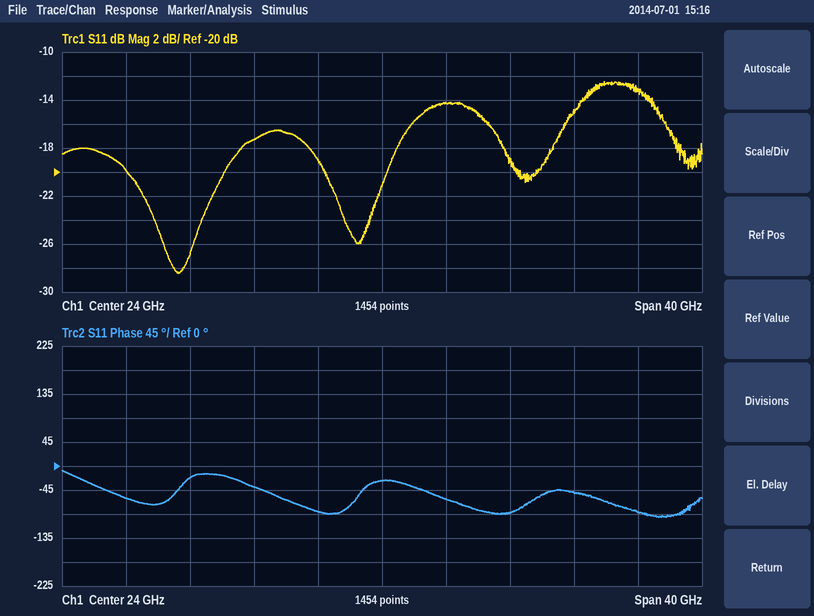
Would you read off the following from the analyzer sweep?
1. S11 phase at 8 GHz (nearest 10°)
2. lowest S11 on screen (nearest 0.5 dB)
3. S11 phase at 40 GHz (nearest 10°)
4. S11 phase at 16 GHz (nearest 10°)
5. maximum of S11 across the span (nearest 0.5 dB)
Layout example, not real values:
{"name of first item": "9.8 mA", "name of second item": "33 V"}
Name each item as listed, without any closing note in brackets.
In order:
{"S11 phase at 8 GHz": "-60°", "lowest S11 on screen": "-28.5 dB", "S11 phase at 40 GHz": "-90°", "S11 phase at 16 GHz": "-40°", "maximum of S11 across the span": "-12.5 dB"}
